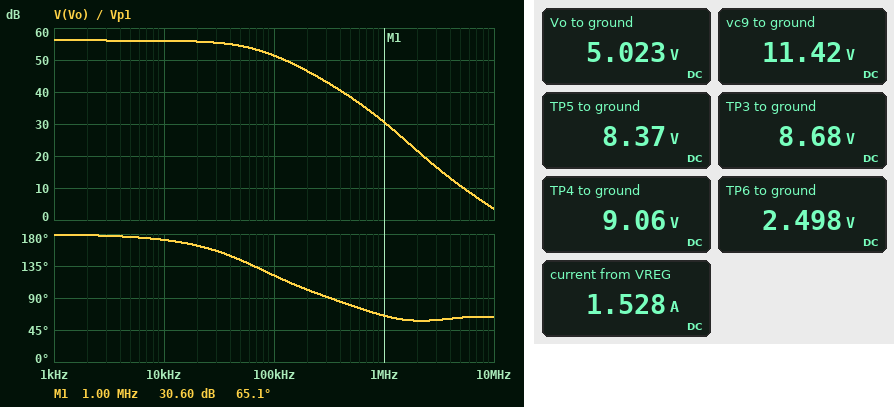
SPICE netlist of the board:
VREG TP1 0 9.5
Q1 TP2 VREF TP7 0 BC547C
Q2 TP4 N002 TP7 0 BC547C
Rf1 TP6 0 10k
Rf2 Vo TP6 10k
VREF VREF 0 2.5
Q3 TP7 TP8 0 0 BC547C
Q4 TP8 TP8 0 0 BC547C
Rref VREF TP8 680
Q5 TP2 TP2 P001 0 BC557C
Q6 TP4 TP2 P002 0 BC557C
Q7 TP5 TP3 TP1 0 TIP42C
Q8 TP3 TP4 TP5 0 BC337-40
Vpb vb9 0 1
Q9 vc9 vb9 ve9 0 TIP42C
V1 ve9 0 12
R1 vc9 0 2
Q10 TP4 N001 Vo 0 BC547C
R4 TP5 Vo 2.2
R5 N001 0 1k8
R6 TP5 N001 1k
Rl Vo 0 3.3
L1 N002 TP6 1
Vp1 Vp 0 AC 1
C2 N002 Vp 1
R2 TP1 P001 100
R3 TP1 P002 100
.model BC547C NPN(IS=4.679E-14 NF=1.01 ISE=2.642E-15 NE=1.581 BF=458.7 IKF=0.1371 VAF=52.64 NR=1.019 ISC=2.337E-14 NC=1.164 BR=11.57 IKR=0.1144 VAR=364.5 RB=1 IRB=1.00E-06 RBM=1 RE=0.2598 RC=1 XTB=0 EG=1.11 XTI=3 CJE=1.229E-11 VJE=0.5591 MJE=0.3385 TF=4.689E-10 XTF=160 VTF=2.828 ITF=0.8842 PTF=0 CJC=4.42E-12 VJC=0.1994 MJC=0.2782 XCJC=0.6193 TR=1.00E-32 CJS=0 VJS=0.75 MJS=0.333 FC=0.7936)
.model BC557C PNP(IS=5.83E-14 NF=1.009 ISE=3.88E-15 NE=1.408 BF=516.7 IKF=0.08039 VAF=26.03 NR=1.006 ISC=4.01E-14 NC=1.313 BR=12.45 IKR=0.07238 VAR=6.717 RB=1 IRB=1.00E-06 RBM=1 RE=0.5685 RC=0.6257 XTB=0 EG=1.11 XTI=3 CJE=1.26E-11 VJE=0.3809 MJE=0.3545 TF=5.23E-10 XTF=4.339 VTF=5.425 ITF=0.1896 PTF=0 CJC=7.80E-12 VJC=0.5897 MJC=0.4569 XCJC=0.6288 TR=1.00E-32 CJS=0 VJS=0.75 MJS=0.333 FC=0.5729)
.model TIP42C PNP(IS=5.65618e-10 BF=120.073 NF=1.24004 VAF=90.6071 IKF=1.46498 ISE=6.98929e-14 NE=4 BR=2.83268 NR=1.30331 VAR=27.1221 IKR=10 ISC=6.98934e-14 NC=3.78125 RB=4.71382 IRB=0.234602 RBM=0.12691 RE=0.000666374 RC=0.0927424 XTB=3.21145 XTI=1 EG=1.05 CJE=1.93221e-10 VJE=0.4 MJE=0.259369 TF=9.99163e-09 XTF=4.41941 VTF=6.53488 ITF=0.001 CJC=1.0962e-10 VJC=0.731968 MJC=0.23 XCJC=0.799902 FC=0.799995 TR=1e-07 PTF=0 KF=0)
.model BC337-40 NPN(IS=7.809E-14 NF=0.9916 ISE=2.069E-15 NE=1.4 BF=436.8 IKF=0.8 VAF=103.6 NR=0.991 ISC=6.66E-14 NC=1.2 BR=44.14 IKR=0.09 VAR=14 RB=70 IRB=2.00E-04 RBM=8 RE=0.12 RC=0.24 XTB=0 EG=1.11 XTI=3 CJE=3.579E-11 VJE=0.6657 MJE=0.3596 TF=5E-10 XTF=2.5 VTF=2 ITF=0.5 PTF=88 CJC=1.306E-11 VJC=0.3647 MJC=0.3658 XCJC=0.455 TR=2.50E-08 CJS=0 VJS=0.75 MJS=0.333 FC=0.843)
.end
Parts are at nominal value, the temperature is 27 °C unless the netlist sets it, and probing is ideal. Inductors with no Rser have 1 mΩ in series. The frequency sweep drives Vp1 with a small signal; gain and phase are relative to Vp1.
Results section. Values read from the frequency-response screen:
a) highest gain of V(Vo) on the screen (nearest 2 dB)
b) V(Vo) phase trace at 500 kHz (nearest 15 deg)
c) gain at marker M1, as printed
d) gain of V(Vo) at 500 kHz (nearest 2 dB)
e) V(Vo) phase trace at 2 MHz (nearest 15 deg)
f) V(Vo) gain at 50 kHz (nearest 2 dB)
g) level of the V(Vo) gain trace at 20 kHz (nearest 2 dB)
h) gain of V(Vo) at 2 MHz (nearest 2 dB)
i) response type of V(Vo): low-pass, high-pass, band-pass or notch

56 dB
75 deg
30.60 dB
38 dB
60 deg
54 dB
56 dB
22 dB
low-pass
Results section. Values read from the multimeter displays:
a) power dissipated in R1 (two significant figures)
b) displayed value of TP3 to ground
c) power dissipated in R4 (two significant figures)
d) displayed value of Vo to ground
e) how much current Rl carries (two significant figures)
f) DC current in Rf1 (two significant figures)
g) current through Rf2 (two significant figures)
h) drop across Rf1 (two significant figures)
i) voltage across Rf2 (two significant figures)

65 W
8.68 V
5.1 W
5.023 V
1.5 A
250 µA
250 µA
2.5 V
2.5 V
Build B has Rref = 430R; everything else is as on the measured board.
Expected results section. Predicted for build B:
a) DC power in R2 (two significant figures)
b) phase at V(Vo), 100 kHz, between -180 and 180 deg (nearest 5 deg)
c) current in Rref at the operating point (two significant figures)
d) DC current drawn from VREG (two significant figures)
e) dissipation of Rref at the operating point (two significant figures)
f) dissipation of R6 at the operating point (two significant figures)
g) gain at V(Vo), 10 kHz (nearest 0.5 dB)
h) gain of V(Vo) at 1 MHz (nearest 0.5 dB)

490 µW
135 deg
4.3 mA
1.5 A
7.9 mW
9.0 mW
55.0 dB
34.0 dB
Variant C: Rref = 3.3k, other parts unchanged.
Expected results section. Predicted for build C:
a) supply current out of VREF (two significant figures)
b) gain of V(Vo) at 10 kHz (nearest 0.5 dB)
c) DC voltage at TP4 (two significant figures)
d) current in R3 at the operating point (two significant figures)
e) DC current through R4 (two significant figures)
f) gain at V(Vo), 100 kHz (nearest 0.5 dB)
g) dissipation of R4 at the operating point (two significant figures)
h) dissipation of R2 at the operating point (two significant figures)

570 µA
48.0 dB
9.0 V
320 µA
1.5 A
40.0 dB
5.0 W
11 µW
